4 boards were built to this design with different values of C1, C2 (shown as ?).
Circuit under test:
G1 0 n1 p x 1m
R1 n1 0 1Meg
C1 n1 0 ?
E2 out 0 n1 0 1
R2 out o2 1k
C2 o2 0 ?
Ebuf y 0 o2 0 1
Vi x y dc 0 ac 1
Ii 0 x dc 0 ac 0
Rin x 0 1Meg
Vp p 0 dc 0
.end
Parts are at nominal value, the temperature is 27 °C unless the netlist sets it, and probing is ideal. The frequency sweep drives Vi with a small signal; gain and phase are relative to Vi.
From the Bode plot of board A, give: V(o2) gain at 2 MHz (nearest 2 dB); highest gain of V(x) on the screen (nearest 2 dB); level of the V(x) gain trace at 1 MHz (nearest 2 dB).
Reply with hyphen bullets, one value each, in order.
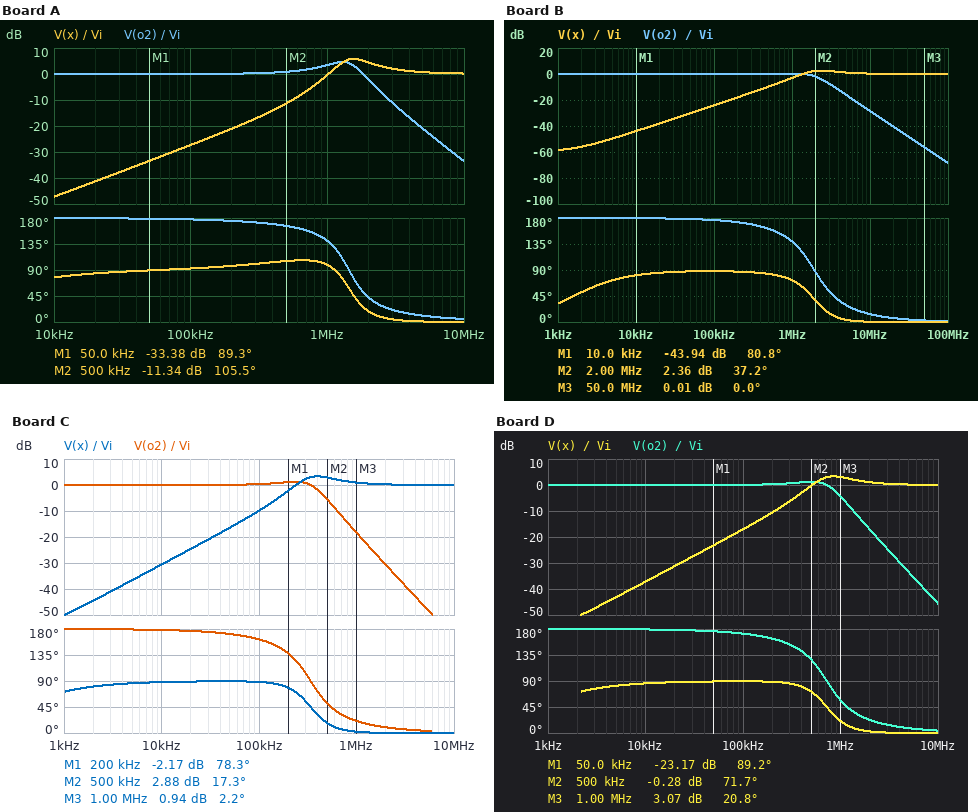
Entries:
- -2 dB
- 6 dB
- 0 dB
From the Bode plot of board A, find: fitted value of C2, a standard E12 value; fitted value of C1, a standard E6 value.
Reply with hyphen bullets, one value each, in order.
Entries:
- 180 pF
- 68 pF
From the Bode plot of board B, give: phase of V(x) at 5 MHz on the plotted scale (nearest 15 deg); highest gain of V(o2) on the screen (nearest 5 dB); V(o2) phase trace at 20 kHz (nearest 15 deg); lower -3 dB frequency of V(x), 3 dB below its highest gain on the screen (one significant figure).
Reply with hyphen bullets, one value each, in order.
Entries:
- 0 deg
- 0 dB
- 180 deg
- 1 MHz
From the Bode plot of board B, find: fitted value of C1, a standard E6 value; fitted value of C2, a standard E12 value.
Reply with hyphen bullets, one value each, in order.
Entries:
- 100 pF
- 68 pF
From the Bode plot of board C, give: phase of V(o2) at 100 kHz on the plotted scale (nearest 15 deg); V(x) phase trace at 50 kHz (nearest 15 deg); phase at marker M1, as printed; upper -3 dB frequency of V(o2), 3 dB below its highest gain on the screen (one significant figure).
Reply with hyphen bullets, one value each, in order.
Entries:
- 165 deg
- 90 deg
- 78.3 deg
- 400 kHz
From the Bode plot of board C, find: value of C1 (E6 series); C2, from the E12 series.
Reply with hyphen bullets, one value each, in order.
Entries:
- 470 pF
- 470 pF
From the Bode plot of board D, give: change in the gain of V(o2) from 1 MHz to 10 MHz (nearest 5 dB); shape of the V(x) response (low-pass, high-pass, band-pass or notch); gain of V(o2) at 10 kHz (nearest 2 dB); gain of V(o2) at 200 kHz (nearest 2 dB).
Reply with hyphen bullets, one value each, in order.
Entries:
- -40 dB
- high-pass
- 0 dB
- 0 dB
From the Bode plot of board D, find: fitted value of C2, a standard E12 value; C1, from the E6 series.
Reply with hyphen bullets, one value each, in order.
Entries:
- 220 pF
- 220 pF
